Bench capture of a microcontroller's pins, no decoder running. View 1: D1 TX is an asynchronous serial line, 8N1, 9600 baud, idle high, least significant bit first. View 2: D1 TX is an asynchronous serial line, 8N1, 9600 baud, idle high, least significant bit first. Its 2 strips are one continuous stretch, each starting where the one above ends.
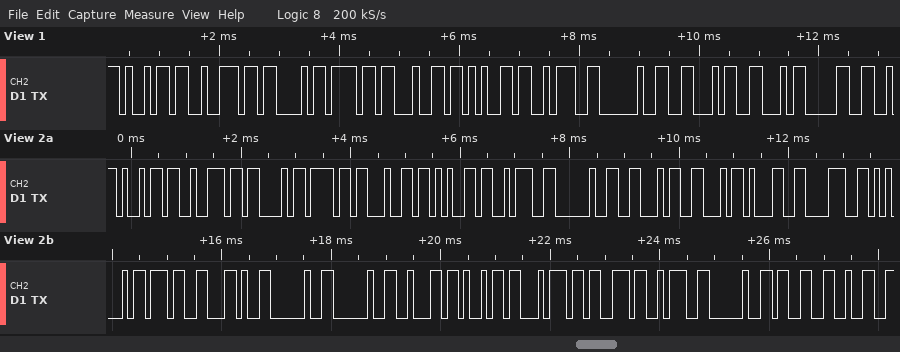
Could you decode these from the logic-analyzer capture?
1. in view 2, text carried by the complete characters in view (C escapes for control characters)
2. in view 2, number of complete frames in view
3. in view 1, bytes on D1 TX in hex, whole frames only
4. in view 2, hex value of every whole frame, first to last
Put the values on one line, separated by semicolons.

"irCode: FF18E7,  bits: 32"; 25; 0x69 0x72 0x43 0x6F 0x64 0x65 0x3A 0x20 0x46 0x46 0x30; 69 72 43 6F 64 65 3A 20 46 46 31 38 45 37 2C 20 20 62 69 74 73 3A 20 33 32
